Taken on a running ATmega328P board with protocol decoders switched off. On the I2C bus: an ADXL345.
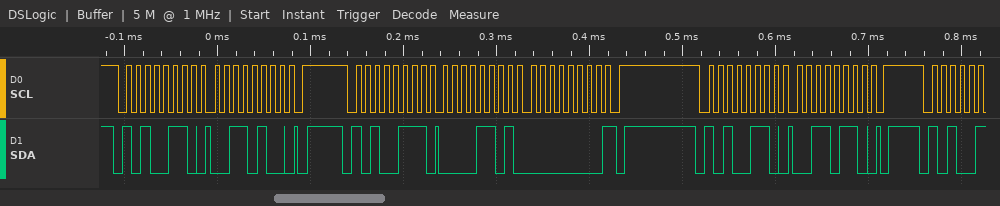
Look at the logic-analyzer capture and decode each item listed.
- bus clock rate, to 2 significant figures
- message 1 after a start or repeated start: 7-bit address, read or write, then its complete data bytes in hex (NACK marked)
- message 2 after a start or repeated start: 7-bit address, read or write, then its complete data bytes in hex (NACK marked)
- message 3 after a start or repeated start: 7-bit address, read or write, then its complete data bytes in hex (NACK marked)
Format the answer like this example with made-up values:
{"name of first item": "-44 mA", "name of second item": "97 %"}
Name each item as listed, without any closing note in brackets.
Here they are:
{"bus clock rate, to 2 significant figures": "100 kHz", "message 1 after a start or repeated start: 7-bit address, read or write, then its complete data bytes in hex": "0x53 write: 34", "message 2 after a start or repeated start: 7-bit address, read or write, then its complete data bytes in hex": "0x53 read: 0D 00 NACK", "message 3 after a start or repeated start: 7-bit address, read or write, then its complete data bytes in hex": "0x53 write: 36"}
